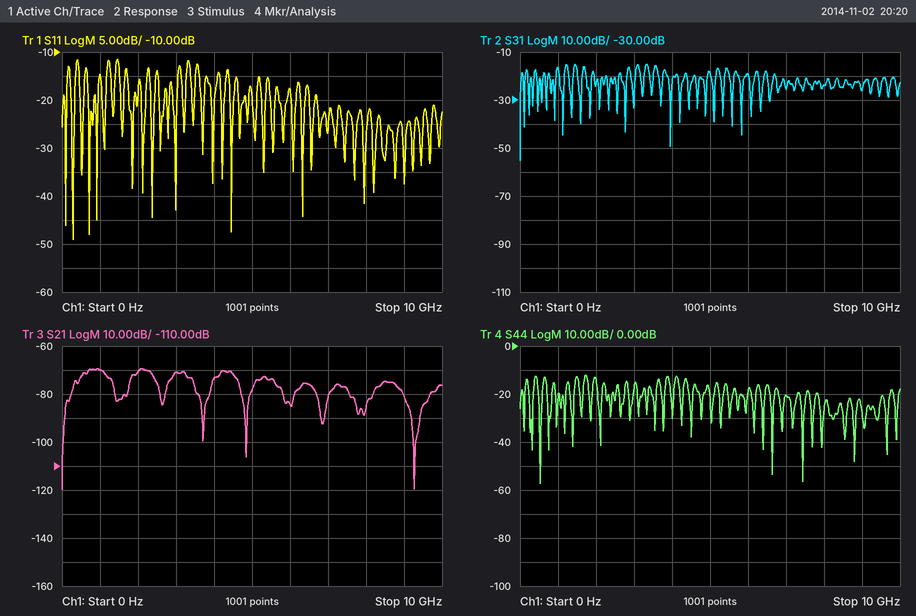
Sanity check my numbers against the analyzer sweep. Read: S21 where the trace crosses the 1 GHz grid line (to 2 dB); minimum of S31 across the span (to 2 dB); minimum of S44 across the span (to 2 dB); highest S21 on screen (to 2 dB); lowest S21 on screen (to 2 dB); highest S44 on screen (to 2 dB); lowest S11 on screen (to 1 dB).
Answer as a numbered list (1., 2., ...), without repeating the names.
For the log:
1. -70 dB
2. -56 dB
3. -58 dB
4. -70 dB
5. -120 dB
6. -12 dB
7. -49 dB
